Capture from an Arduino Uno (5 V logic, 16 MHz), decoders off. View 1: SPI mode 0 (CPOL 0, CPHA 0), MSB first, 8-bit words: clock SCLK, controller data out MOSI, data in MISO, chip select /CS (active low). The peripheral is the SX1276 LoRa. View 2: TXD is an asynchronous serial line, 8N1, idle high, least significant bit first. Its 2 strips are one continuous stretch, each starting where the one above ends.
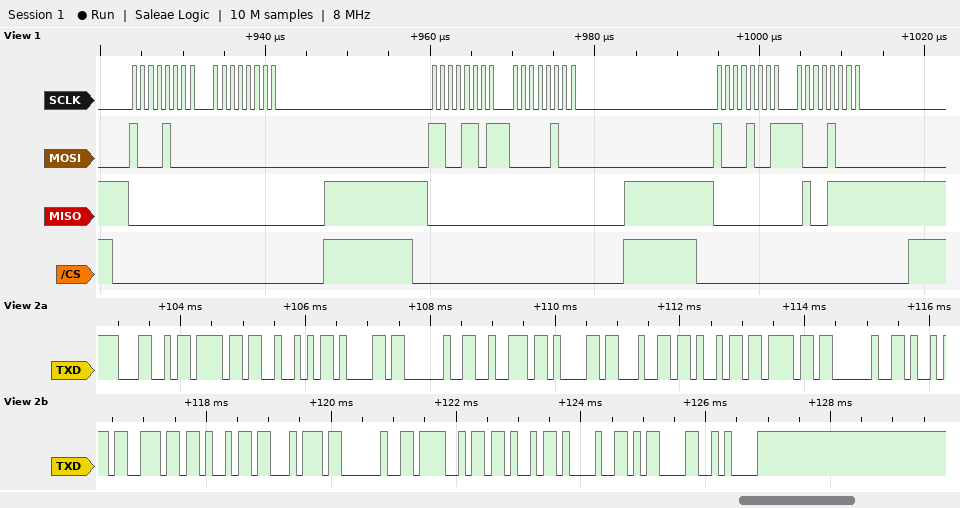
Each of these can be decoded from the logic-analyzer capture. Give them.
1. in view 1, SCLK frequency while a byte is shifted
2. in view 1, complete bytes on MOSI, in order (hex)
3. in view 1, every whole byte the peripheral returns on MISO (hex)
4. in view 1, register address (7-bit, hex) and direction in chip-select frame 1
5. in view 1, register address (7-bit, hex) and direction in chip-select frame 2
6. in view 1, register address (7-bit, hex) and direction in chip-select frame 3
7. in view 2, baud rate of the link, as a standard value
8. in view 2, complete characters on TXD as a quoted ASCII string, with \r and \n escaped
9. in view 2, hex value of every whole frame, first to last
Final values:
1 MHz
88 00 CD 04 89 88
00 00 00 00 00 4F
0x08 write
0x4D write
0x09 write
9600 baud
"LoRa radio init OK!\r\n"
4C 6F 52 61 20 72 61 64 69 6F 20 69 6E 69 74 20 4F 4B 21 0D 0A
